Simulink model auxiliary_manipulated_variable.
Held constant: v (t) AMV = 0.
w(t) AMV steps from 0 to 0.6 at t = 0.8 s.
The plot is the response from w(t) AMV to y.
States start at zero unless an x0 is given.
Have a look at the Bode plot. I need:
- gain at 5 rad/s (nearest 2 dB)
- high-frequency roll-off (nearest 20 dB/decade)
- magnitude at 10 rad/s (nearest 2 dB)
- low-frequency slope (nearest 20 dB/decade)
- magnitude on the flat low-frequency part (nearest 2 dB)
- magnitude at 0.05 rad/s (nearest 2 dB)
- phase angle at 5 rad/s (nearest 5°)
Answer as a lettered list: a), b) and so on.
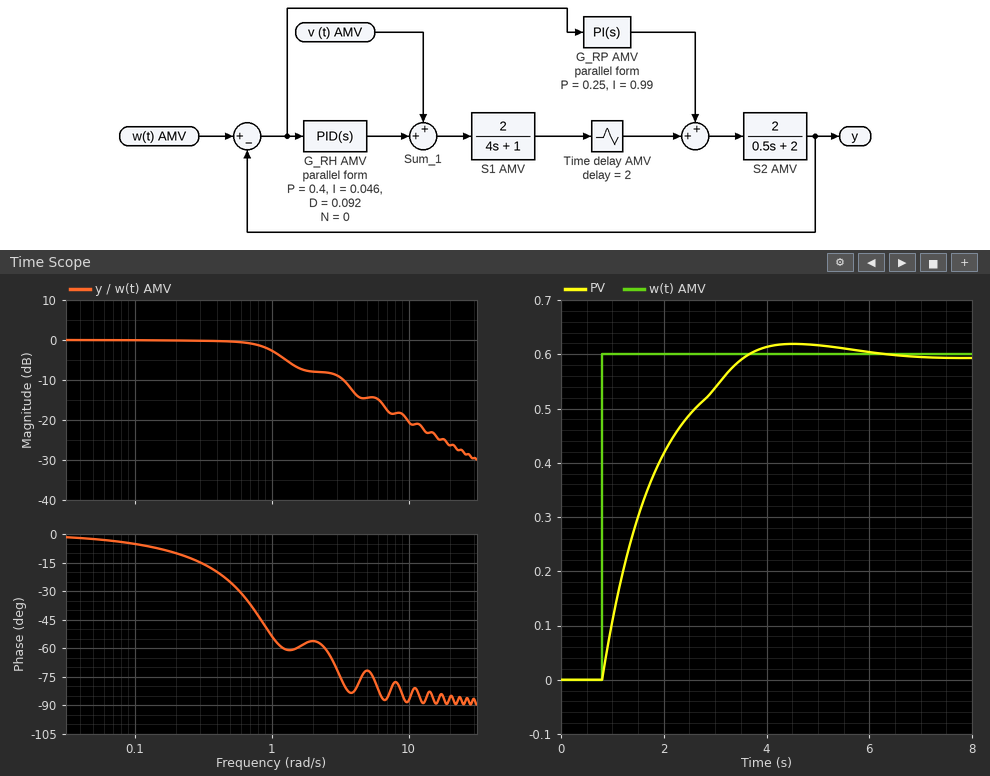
a) -14 dB
b) -20 dB/decade
c) -20 dB
d) 0 dB/decade
e) 0 dB
f) 0 dB
g) -70°
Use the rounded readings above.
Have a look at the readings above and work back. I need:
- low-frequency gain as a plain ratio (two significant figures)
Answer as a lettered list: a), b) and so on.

a) 1.0
